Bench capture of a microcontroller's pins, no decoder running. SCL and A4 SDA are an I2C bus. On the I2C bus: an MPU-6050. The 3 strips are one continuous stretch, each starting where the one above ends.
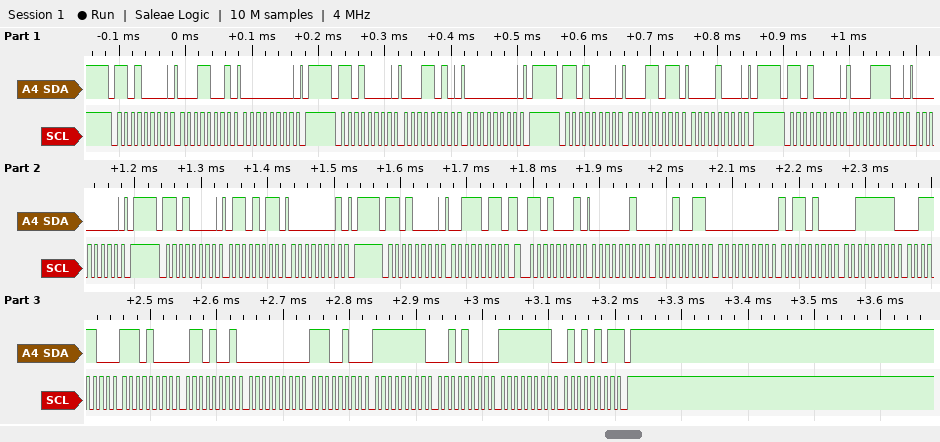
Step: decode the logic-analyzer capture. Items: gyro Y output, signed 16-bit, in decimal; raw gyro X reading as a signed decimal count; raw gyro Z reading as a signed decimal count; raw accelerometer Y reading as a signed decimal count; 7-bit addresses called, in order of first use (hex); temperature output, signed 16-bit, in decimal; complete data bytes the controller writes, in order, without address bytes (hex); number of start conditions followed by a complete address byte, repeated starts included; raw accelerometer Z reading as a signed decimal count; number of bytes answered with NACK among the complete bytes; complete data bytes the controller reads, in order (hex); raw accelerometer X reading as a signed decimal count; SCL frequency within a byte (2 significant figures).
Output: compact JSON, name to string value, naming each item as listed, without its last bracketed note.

{"gyro Y output, signed 16-bit, in decimal": "-216", "raw gyro X reading as a signed decimal count": "228", "raw gyro Z reading as a signed decimal count": "-171", "raw accelerometer Y reading as a signed decimal count": "180", "7-bit addresses called, in order of first use": "0x68", "temperature output, signed 16-bit, in decimal": "-6039", "complete data bytes the controller writes, in order, without address bytes": "19 00 1A 00 1B 08 1C 00 6B 01 3B", "number of start conditions followed by a complete address byte, repeated starts included": "7", "raw accelerometer Z reading as a signed decimal count": "16188", "number of bytes answered with NACK among the complete bytes": "1", "complete data bytes the controller reads, in order": "02 13 00 B4 3F 3C E8 69 00 E4 FF 28 FF 55", "raw accelerometer X reading as a signed decimal count": "531", "SCL frequency within a byte": "100 kHz"}
